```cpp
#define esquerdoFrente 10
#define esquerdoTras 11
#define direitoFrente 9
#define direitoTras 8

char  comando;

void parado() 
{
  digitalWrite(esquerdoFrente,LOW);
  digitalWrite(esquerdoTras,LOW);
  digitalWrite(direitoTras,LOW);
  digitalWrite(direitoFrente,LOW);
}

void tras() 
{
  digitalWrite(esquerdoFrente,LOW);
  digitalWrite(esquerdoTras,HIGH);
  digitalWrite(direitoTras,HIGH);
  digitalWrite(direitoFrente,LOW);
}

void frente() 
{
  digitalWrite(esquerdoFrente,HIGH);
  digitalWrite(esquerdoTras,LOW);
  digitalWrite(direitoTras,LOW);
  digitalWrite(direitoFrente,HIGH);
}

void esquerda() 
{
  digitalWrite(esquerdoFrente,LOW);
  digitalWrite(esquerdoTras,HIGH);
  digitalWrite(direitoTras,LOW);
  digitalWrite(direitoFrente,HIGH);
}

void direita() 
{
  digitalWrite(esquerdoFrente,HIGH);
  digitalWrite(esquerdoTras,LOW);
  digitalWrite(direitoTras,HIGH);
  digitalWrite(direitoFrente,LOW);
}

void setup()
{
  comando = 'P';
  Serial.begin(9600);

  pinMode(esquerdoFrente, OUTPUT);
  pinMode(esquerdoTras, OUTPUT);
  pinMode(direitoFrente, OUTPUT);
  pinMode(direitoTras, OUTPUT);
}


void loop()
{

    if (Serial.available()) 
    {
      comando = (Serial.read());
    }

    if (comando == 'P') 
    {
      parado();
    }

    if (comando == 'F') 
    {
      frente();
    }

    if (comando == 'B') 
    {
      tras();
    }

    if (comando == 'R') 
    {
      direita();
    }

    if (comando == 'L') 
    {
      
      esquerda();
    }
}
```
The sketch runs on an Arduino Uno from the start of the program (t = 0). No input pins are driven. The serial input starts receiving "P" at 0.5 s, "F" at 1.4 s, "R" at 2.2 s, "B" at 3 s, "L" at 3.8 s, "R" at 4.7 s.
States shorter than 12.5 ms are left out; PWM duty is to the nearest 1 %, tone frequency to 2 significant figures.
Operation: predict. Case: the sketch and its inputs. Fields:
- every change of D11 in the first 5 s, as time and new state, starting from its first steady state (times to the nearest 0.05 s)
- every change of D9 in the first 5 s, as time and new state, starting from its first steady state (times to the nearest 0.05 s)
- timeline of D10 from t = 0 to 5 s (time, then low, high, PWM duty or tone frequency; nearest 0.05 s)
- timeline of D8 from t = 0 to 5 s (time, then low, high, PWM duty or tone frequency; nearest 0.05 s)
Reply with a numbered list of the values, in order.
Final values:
1. 0 s low; 3 s high; 4.7 s low
2. 0 s low; 1.4 s high; 2.2 s low; 3.8 s high; 4.7 s low
3. 0 s low; 1.4 s high; 3 s low; 4.7 s high
4. 0 s low; 2.2 s high; 3.8 s low; 4.7 s high
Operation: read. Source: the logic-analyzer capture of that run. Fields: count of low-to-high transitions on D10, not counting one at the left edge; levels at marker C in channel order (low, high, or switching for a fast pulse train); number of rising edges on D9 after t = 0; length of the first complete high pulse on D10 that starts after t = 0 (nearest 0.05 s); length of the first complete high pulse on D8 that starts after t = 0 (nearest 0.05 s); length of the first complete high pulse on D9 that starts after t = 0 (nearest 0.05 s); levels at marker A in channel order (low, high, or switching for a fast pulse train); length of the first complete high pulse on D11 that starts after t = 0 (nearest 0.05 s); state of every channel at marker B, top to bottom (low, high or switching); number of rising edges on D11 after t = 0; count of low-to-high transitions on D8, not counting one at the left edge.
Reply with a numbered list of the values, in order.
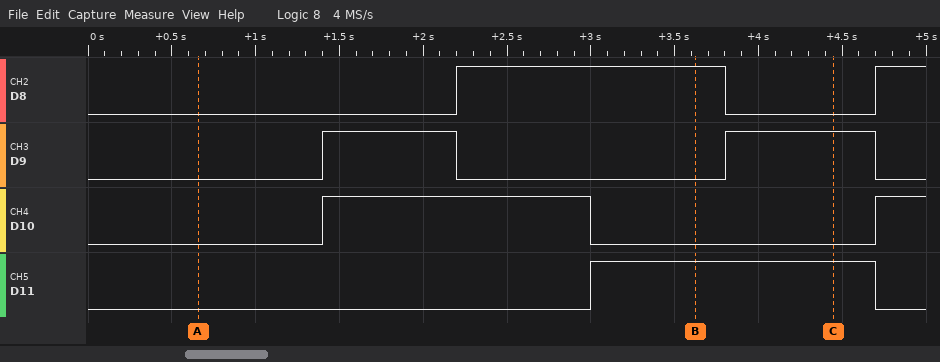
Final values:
1. 2
2. D8 low, D9 high, D10 low, D11 high
3. 2
4. 1.60 s
5. 1.60 s
6. 0.80 s
7. D8 low, D9 low, D10 low, D11 low
8. 1.70 s
9. D8 high, D9 low, D10 low, D11 high
10. 1
11. 2
